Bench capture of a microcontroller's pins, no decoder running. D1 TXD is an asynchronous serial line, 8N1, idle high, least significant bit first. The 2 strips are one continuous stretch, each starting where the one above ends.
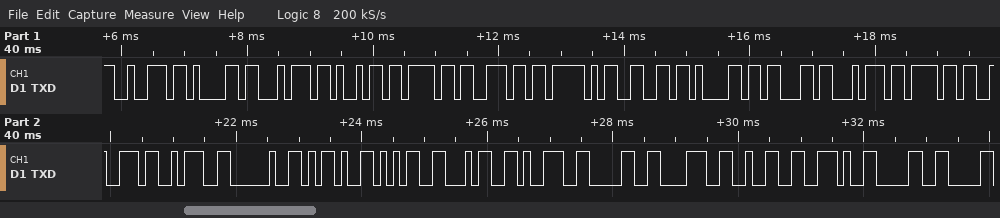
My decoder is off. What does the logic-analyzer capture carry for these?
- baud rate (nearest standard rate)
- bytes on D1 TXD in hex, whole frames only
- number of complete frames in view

9600 baud
72 61 74 69 6F 6E 5F 66 61 63 74 6F 72 3A 20 2D 35 34 39 30 38 32 2E 30
24
